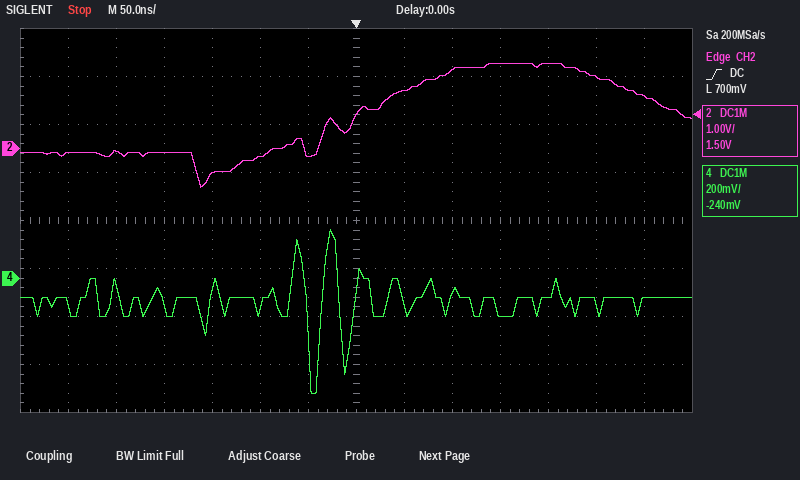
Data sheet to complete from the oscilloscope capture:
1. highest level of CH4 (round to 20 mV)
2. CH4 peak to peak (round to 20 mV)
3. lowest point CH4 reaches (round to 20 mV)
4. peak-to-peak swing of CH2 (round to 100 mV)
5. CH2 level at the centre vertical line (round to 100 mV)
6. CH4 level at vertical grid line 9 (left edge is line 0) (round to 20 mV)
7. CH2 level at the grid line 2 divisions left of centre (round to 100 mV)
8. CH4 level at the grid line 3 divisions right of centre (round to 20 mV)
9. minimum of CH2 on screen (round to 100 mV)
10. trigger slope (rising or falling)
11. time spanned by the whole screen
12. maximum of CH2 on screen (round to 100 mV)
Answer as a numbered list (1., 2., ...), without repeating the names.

1. 200 mV
2. 680 mV
3. -480 mV
4. 2.6 V
5. 700 mV
6. -60 mV
7. -200 mV
8. -160 mV
9. -800 mV
10. rising
11. 700 ns
12. 1.8 V
